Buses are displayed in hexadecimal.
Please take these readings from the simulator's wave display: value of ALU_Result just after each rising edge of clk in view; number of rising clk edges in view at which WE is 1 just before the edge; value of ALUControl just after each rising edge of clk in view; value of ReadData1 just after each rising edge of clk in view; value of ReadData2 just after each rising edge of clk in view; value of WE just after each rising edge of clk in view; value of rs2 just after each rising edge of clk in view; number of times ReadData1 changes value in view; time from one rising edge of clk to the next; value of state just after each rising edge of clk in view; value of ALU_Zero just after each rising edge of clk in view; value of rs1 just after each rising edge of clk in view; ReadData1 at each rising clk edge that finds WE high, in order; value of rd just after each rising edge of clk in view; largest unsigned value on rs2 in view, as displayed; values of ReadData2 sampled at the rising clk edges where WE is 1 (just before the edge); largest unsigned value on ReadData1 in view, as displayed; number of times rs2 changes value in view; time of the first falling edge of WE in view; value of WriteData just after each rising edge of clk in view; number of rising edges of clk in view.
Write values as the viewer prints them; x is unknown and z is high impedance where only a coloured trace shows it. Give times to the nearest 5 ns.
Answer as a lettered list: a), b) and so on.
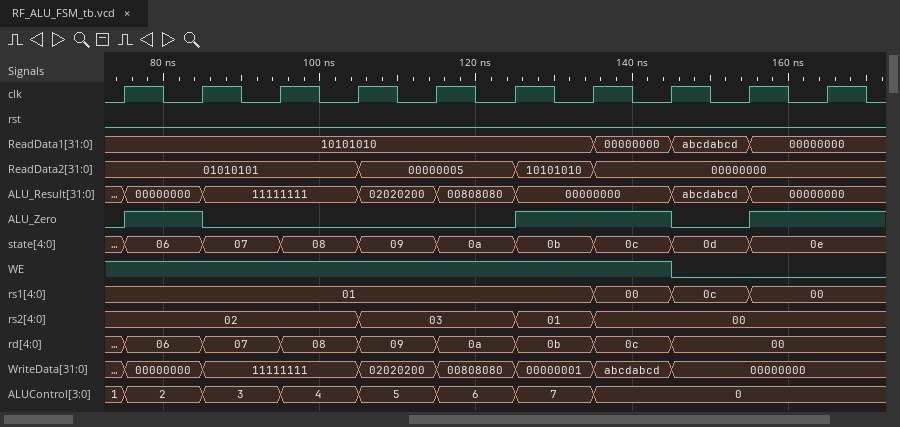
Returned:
a) 00000000, 11111111, 11111111, 02020200, 00808080, 00000000, 00000000, abcdabcd, 00000000, 00000000
b) 8
c) 2, 3, 4, 5, 6, 7, 0, 0, 0, 0
d) 10101010, 10101010, 10101010, 10101010, 10101010, 10101010, 00000000, abcdabcd, 00000000, 00000000
e) 01010101, 01010101, 01010101, 00000005, 00000005, 10101010, 00000000, 00000000, 00000000, 00000000
f) 1 1 1 1 1 1 1 0 0 0
g) 02, 02, 02, 03, 03, 01, 00, 00, 00, 00
h) 3
i) 10 ns
j) 06, 07, 08, 09, 0a, 0b, 0c, 0d, 0e, 0e
k) 1 0 0 0 0 1 1 0 1 1
l) 01, 01, 01, 01, 01, 01, 00, 0c, 00, 00
m) 10101010, 10101010, 10101010, 10101010, 10101010, 10101010, 10101010, 00000000
n) 06, 07, 08, 09, 0a, 0b, 0c, 00, 00, 00
o) 03
p) 01010101, 01010101, 01010101, 01010101, 00000005, 00000005, 10101010, 00000000
q) abcdabcd
r) 3
s) 145 ns
t) 00000000, 11111111, 11111111, 02020200, 00808080, 00000001, abcdabcd, 00000000, 00000000, 00000000
u) 10
